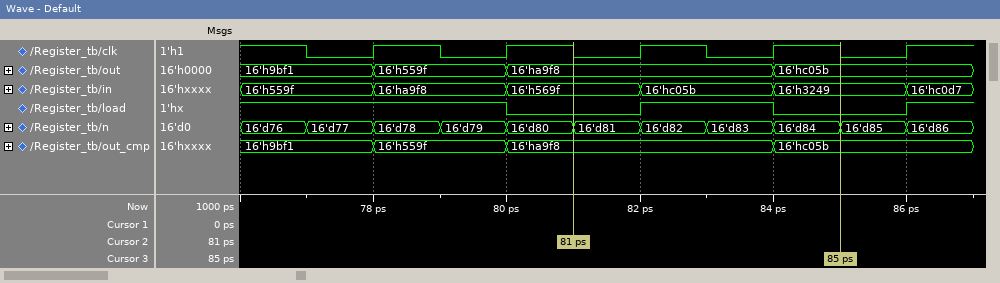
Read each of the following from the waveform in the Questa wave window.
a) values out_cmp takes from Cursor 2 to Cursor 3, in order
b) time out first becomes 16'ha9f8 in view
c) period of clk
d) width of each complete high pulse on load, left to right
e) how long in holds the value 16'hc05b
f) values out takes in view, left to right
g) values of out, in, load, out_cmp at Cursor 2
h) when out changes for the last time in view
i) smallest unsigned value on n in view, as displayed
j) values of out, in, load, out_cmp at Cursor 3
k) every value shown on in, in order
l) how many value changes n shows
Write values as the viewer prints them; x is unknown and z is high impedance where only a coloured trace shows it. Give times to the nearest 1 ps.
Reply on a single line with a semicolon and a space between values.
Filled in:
16'ha9f8, 16'hc05b; 80 ps; 2 ps; 2 ps; 2 ps; 16'h9bf1, 16'h559f, 16'ha9f8, 16'hc05b; out=16'ha9f8, in=16'h569f, load=0, out_cmp=16'ha9f8; 84 ps; 16'd76; out=16'hc05b, in=16'h3249, load=0, out_cmp=16'hc05b; 16'h559f, 16'ha9f8, 16'h569f, 16'hc05b, 16'h3249, 16'hc0d7; 10
